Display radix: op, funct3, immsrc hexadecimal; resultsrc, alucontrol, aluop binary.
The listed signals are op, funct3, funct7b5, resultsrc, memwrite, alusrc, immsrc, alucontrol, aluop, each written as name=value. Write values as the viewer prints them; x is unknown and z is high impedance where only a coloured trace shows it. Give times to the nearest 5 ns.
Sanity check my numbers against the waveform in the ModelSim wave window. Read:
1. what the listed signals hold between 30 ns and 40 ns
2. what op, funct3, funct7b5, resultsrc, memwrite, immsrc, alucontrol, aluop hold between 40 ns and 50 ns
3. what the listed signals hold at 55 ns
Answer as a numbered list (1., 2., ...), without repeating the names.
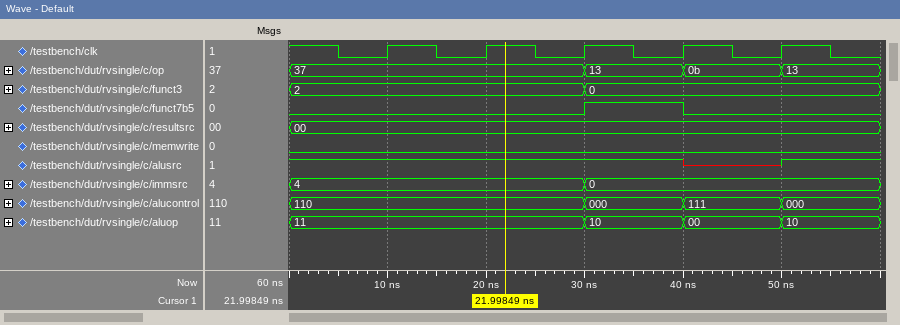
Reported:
1. op=13, funct3=0, funct7b5=1, resultsrc=00, memwrite=0, alusrc=1, immsrc=0, alucontrol=000, aluop=10
2. op=0b, funct3=0, funct7b5=0, resultsrc=00, memwrite=0, immsrc=0, alucontrol=111, aluop=00
3. op=13, funct3=0, funct7b5=0, resultsrc=00, memwrite=0, alusrc=1, immsrc=0, alucontrol=000, aluop=10
